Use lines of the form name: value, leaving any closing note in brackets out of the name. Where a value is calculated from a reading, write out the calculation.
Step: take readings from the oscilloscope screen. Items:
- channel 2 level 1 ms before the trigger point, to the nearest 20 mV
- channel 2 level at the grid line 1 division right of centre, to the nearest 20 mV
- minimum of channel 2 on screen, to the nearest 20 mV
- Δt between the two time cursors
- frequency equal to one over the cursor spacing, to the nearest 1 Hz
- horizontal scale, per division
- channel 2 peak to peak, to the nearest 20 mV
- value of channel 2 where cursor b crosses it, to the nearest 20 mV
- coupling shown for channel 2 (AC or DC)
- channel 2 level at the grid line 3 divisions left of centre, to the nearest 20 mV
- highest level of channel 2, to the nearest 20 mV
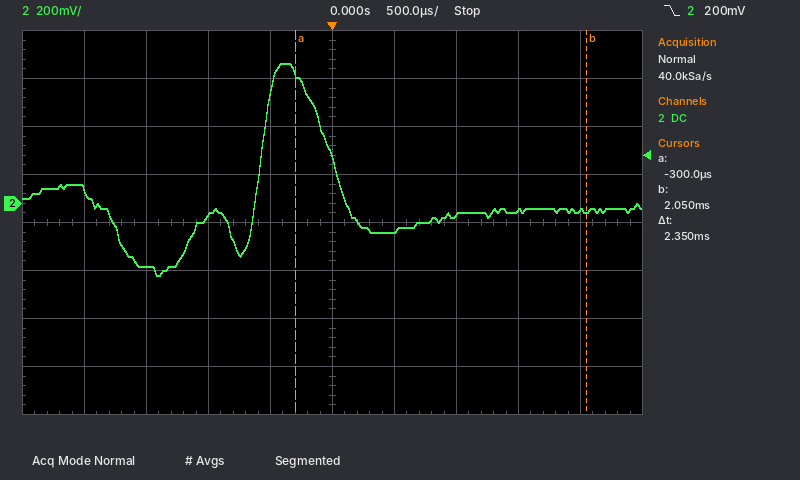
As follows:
channel 2 level 1 ms before the trigger point, to the nearest 20 mV: -60 mV
channel 2 level at the grid line 1 division right of centre, to the nearest 20 mV: -120 mV
minimum of channel 2 on screen, to the nearest 20 mV: -300 mV
Δt between the two time cursors: 2.35 ms
frequency equal to one over the cursor spacing, to the nearest 1 Hz: 1 / 2.35 ms ≈ 426 Hz
horizontal scale, per division: 500 µs
channel 2 peak to peak, to the nearest 20 mV: 580 mV − (-300 mV) = 880 mV
value of channel 2 where cursor b crosses it, to the nearest 20 mV: -40 mV
coupling shown for channel 2: DC
channel 2 level at the grid line 3 divisions left of centre, to the nearest 20 mV: -260 mV
highest level of channel 2, to the nearest 20 mV: 580 mV
